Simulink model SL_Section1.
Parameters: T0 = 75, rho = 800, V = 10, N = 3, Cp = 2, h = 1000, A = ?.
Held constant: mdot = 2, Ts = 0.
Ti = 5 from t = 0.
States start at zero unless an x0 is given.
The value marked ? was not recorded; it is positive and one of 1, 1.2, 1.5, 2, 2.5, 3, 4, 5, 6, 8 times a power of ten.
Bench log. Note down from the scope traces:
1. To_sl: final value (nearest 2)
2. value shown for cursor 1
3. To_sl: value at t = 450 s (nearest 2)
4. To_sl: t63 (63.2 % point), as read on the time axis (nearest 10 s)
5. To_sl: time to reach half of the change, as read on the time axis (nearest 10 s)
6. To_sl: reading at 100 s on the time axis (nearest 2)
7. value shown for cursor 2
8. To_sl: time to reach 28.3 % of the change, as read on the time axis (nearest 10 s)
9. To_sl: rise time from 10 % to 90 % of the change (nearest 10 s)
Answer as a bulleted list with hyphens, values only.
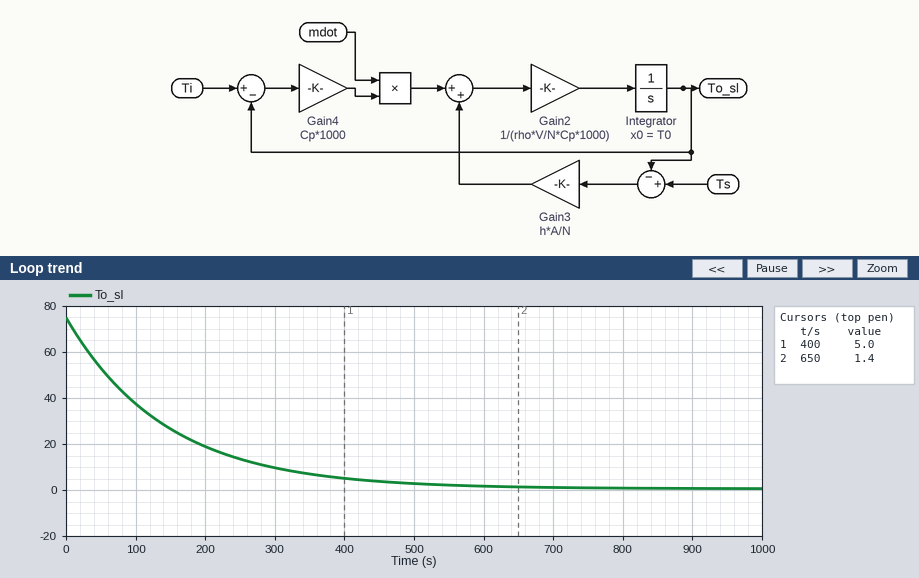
- 0
- 5.0
- 4
- 140 s
- 100 s
- 38
- 1.4
- 50 s
- 310 s
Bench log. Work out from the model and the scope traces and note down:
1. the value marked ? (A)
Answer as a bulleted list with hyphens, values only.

- 100
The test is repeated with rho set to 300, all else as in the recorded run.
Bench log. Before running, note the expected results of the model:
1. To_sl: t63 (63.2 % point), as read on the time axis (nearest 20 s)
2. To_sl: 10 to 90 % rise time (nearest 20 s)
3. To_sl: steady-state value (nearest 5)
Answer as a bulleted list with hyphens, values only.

- 60 s
- 120 s
- 0
